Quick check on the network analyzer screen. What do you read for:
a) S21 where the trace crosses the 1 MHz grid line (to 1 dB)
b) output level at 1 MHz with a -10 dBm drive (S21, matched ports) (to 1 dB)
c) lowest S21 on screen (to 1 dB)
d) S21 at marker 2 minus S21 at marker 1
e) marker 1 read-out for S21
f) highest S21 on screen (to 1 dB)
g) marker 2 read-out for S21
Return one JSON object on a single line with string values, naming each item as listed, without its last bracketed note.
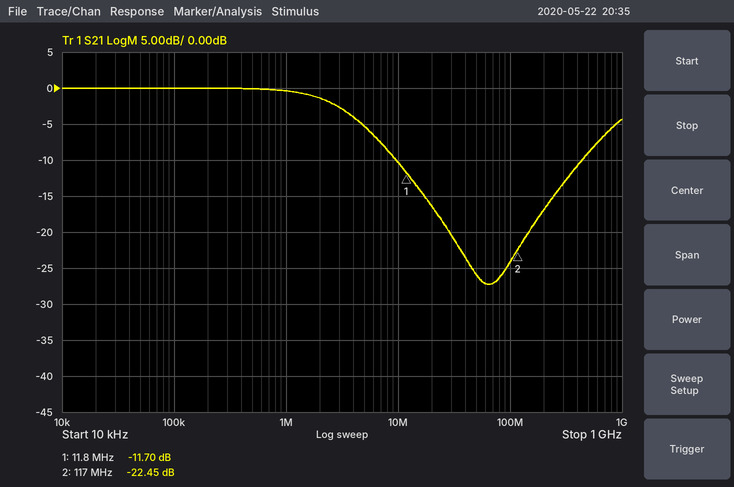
{"S21 where the trace crosses the 1 MHz grid line": "0 dB", "output level at 1 MHz with a -10 dBm drive (S21, matched ports)": "-10 dBm", "lowest S21 on screen": "-27 dB", "S21 at marker 2 minus S21 at marker 1": "-10.75 dB", "marker 1 read-out for S21": "-11.70 dB", "highest S21 on screen": "0 dB", "marker 2 read-out for S21": "-22.45 dB"}
